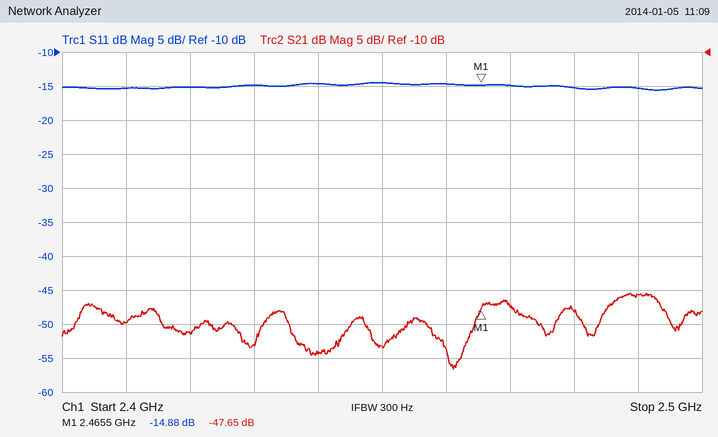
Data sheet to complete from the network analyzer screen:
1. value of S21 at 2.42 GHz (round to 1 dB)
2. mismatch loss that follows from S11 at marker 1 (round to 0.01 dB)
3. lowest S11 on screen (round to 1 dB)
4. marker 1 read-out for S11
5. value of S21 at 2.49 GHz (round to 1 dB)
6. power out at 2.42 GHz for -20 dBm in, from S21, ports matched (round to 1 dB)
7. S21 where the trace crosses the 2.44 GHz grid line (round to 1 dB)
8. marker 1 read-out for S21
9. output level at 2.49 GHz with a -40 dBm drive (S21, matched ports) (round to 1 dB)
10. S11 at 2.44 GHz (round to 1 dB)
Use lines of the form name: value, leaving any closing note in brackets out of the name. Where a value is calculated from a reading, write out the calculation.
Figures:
value of S21 at 2.42 GHz: -51 dB
mismatch loss that follows from S11 at marker 1: −10 log10(1 − 10^(-14.88/10)) ≈ 0.14 dB
lowest S11 on screen: -16 dB
marker 1 read-out for S11: -14.88 dB
value of S21 at 2.49 GHz: -46 dB
power out at 2.42 GHz for -20 dBm in, from S21, ports matched: -20 dBm + (-51 dB) = -71 dBm
S21 where the trace crosses the 2.44 GHz grid line: -54 dB
marker 1 read-out for S21: -47.65 dB
output level at 2.49 GHz with a -40 dBm drive (S21, matched ports): -40 dBm + (-46 dB) = -86 dBm
S11 at 2.44 GHz: -15 dB
